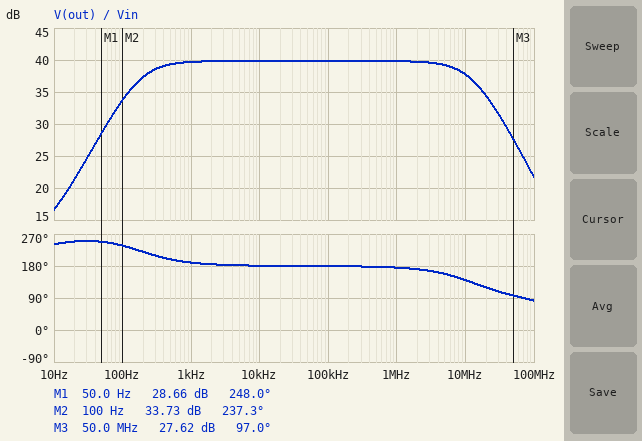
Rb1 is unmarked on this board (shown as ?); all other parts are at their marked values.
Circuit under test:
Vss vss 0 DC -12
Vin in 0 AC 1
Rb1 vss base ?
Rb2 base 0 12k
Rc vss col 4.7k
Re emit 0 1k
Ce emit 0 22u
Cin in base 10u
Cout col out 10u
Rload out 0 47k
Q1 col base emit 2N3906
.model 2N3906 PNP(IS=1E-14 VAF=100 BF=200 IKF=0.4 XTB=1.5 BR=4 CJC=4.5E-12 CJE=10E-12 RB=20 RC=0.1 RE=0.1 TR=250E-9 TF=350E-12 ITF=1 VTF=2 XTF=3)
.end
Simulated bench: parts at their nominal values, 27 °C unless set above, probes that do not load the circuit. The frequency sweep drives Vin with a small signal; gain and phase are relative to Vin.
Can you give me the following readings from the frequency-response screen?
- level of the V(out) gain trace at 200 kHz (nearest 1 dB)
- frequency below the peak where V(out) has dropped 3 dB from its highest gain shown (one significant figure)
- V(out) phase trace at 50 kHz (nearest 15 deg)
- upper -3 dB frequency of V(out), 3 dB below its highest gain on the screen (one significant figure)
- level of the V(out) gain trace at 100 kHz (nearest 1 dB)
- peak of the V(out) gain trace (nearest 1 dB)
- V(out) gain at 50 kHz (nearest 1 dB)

40 dB
200 Hz
180 deg
10 MHz
40 dB
40 dB
40 dB
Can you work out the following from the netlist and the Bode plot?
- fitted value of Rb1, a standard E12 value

100 kΩ
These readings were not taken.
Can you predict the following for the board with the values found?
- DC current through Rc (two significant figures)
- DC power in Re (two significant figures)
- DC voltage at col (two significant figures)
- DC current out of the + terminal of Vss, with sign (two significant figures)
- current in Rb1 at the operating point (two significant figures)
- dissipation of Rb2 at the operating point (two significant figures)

610 µA
380 µW
-9.1 V
-720 µA
110 µA
130 µW
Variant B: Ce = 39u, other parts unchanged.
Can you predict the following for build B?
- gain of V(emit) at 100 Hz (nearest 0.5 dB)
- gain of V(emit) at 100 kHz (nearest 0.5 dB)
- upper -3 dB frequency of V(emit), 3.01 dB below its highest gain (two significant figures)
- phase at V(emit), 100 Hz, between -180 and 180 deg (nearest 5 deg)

-3.5 dB
-60.5 dB
100 Hz
-45 deg
